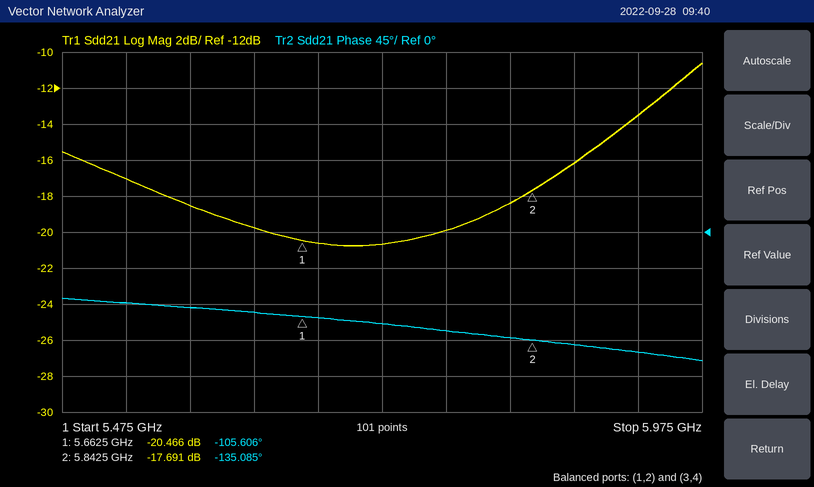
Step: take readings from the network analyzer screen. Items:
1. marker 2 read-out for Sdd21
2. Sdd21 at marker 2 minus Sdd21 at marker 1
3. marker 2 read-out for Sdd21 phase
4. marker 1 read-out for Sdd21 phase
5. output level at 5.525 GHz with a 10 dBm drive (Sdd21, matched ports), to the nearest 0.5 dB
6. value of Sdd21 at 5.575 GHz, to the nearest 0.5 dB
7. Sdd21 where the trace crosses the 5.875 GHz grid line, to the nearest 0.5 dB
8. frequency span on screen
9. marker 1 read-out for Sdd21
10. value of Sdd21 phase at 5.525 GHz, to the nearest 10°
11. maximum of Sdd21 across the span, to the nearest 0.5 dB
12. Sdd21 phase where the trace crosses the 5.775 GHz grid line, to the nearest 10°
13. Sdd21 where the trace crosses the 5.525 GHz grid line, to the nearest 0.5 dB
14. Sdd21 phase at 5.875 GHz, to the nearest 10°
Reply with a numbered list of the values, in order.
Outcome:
1. -17.691 dB
2. 2.775 dB
3. -135.085°
4. -105.606°
5. -7.0 dBm
6. -18.5 dB
7. -16.0 dB
8. 500 MHz
9. -20.466 dB
10. -90°
11. -10.5 dB
12. -120°
13. -17.0 dB
14. -140°
